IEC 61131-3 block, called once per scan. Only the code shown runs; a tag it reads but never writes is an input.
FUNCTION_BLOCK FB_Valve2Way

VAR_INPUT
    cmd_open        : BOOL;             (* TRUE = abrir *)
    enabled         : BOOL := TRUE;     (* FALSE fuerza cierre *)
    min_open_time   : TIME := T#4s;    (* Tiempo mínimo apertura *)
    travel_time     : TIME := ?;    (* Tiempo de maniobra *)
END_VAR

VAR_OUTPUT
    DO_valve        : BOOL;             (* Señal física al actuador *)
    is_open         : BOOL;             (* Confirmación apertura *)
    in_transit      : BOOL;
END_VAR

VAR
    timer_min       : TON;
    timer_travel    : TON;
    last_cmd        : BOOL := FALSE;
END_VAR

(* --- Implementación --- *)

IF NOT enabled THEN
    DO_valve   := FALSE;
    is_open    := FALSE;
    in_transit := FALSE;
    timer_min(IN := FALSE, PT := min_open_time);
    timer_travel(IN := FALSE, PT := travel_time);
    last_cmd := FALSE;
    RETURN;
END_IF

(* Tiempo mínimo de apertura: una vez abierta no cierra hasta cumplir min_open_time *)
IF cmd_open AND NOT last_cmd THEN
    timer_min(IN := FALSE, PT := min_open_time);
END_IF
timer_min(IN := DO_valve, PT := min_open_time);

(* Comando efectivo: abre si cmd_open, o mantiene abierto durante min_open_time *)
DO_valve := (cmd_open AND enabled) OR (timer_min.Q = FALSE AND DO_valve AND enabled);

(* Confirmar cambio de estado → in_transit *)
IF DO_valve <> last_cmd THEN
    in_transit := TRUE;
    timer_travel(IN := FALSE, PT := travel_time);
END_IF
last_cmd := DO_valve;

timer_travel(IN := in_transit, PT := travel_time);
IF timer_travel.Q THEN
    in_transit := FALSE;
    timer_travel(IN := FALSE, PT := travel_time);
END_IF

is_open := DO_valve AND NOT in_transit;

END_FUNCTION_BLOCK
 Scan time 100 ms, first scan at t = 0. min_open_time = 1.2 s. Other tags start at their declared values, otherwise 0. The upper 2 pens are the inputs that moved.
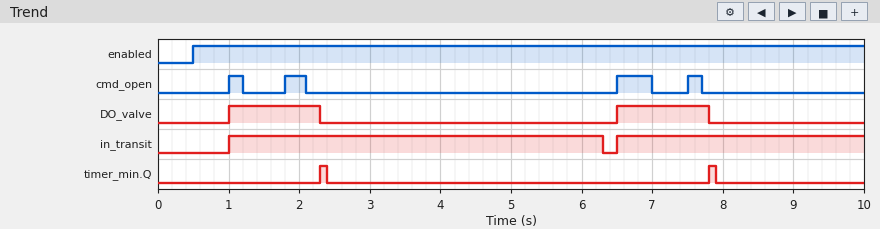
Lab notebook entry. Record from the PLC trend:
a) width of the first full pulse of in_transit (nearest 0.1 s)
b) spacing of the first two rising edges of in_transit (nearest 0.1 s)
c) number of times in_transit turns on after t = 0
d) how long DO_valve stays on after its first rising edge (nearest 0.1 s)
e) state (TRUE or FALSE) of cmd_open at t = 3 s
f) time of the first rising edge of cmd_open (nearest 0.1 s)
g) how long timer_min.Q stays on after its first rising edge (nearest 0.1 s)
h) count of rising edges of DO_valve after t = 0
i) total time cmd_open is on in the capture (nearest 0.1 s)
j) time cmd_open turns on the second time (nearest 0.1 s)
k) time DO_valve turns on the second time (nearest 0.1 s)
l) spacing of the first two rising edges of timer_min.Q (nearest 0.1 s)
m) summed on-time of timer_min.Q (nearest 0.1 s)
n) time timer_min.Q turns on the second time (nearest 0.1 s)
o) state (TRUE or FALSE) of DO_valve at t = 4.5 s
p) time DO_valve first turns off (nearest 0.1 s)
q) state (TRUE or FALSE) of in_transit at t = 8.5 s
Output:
5.3 s
5.5 s
2
1.3 s
FALSE
1.0 s
0.1 s
2
1.2 s
1.8 s
6.5 s
5.5 s
0.2 s
7.8 s
FALSE
2.3 s
TRUE
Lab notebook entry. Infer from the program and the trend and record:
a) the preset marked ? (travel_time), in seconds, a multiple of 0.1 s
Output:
4.0 s
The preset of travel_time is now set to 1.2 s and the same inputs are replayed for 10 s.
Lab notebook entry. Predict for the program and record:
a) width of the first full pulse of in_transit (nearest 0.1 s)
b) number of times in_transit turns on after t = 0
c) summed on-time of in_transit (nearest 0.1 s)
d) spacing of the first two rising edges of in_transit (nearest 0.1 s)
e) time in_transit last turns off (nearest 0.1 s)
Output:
1.2 s
4
4.8 s
1.3 s
9.0 s
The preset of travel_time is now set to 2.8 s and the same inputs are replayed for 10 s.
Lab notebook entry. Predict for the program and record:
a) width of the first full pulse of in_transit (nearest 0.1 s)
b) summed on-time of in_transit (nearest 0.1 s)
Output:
4.1 s
7.6 s
